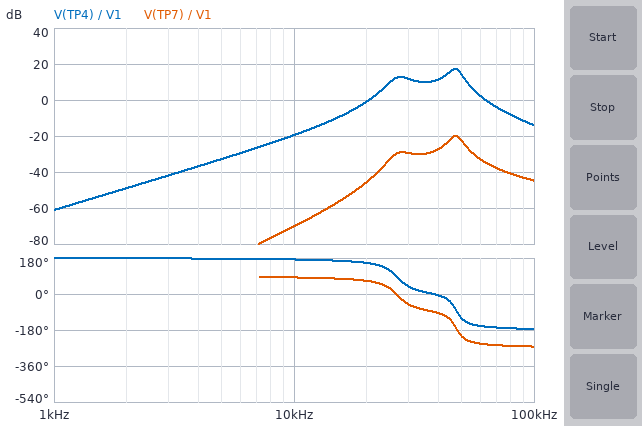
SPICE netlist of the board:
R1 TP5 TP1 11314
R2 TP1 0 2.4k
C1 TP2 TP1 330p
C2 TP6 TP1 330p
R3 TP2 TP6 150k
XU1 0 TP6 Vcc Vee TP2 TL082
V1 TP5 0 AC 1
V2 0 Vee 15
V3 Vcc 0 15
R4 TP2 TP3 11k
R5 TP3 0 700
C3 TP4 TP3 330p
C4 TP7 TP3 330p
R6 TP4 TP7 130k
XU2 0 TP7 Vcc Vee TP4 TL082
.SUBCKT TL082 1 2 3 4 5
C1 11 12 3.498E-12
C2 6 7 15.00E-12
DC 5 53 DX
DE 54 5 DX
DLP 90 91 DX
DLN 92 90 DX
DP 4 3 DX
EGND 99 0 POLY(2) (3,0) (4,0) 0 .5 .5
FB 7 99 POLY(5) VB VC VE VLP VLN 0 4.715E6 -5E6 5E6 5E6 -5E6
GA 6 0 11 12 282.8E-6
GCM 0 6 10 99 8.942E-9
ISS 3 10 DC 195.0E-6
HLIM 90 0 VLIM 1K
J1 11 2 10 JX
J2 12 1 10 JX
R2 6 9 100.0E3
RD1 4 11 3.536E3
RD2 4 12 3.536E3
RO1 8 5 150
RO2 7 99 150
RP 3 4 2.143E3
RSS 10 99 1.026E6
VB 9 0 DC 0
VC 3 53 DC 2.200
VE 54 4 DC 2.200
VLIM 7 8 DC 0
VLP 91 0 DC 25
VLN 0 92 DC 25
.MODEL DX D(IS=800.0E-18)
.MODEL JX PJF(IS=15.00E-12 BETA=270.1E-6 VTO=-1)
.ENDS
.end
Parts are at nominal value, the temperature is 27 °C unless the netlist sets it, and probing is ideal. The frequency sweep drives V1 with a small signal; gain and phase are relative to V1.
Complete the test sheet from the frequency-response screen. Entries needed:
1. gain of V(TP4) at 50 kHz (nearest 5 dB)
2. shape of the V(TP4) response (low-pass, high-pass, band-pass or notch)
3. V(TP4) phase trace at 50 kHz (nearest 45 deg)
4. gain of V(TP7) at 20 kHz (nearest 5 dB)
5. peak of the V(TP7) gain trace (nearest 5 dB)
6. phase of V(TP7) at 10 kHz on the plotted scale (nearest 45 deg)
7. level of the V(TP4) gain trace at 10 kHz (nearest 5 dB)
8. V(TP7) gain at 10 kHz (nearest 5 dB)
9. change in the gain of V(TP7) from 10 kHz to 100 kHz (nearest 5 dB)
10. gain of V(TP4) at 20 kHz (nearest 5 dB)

15 dB
band-pass
-135 deg
-45 dB
-20 dB
90 deg
-20 dB
-70 dB
25 dB
0 dB
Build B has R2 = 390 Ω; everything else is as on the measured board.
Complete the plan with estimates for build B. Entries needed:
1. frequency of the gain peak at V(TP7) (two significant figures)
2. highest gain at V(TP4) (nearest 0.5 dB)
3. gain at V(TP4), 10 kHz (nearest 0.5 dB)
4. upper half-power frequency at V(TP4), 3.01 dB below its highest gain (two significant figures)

54 kHz
24.5 dB
-35.0 dB
56 kHz
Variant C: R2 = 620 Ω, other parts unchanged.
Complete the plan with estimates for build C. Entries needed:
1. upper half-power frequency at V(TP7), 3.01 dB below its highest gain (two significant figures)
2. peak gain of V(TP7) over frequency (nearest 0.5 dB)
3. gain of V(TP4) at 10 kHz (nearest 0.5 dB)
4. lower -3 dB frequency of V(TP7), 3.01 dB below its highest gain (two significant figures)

49 kHz
-5.5 dB
-31.0 dB
45 kHz
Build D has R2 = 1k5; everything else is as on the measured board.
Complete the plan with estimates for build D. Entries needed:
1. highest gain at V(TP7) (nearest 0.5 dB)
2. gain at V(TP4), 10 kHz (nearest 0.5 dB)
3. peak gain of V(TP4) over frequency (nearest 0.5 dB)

-18.0 dB
-23.5 dB
19.0 dB
